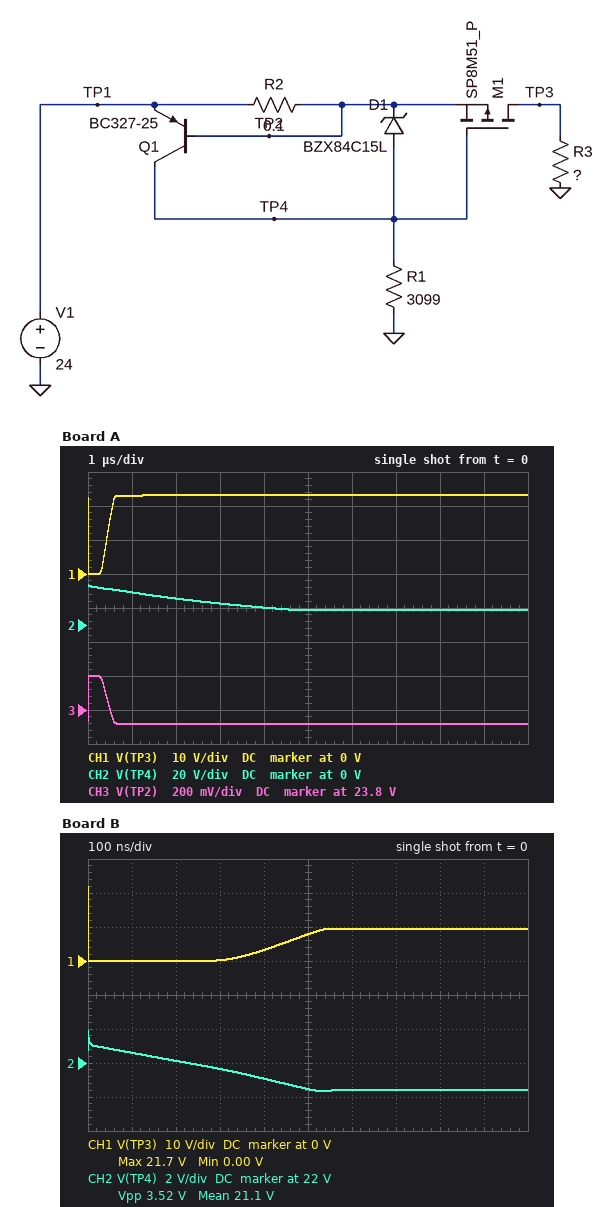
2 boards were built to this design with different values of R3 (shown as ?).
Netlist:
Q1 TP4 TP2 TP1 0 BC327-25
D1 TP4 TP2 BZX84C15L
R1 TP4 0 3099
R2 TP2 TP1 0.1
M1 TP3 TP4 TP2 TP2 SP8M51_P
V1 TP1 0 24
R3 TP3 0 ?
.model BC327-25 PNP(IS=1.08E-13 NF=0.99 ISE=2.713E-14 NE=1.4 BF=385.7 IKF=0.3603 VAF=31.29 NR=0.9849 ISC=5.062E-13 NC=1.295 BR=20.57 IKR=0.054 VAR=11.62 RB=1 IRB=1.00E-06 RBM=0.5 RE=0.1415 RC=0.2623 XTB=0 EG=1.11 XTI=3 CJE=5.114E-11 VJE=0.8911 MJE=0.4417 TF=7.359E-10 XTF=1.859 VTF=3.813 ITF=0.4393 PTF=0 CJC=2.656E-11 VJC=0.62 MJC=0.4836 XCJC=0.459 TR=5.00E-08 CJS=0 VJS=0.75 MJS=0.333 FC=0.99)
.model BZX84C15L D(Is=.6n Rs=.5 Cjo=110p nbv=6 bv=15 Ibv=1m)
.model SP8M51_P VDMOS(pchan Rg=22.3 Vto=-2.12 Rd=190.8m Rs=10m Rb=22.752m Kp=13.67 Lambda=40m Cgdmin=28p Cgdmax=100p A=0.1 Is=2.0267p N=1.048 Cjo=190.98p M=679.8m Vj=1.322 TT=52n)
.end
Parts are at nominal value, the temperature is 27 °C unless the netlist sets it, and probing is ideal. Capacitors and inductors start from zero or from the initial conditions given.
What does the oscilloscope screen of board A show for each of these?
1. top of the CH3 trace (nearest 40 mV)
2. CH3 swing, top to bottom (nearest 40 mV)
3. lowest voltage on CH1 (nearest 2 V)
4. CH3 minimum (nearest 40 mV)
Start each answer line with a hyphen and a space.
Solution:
- 24.00 V
- 280 mV
- 0 V
- 23.72 V
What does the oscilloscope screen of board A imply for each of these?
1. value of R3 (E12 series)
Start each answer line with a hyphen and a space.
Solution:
- 8.2 Ω
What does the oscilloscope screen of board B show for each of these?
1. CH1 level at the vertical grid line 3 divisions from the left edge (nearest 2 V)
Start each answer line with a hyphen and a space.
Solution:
- 0 V
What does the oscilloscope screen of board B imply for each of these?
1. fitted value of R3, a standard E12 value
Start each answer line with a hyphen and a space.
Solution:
- 1.5 Ω
